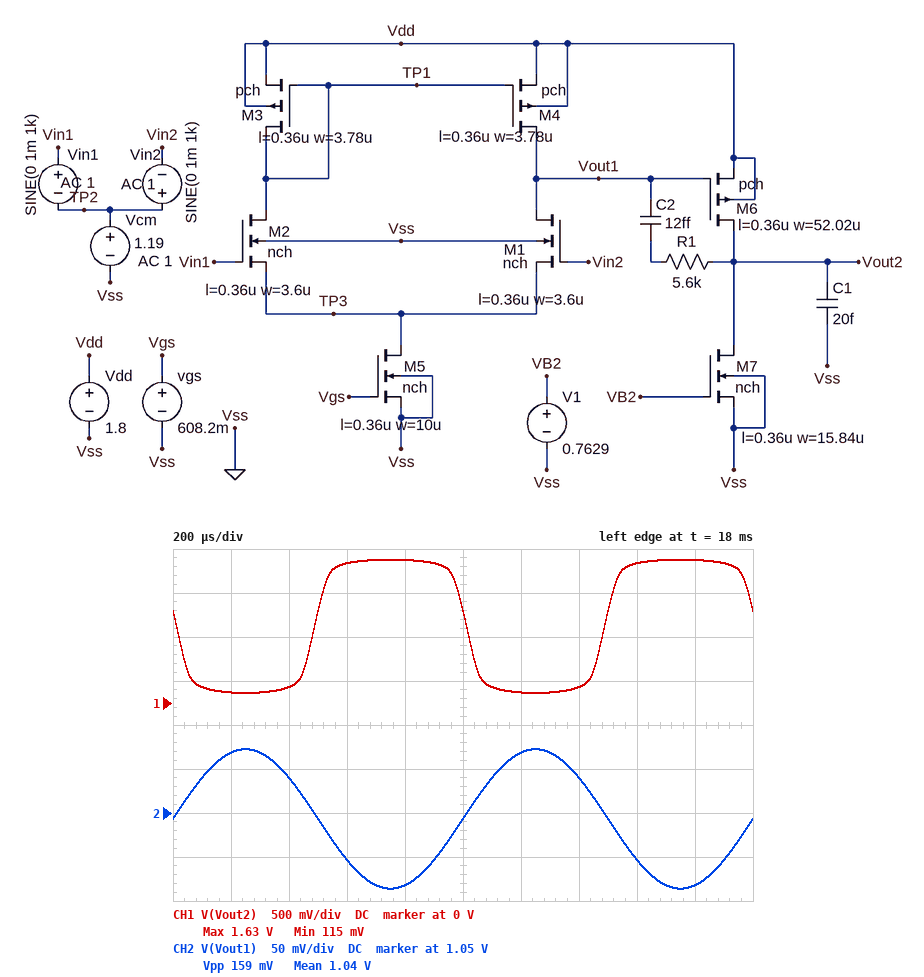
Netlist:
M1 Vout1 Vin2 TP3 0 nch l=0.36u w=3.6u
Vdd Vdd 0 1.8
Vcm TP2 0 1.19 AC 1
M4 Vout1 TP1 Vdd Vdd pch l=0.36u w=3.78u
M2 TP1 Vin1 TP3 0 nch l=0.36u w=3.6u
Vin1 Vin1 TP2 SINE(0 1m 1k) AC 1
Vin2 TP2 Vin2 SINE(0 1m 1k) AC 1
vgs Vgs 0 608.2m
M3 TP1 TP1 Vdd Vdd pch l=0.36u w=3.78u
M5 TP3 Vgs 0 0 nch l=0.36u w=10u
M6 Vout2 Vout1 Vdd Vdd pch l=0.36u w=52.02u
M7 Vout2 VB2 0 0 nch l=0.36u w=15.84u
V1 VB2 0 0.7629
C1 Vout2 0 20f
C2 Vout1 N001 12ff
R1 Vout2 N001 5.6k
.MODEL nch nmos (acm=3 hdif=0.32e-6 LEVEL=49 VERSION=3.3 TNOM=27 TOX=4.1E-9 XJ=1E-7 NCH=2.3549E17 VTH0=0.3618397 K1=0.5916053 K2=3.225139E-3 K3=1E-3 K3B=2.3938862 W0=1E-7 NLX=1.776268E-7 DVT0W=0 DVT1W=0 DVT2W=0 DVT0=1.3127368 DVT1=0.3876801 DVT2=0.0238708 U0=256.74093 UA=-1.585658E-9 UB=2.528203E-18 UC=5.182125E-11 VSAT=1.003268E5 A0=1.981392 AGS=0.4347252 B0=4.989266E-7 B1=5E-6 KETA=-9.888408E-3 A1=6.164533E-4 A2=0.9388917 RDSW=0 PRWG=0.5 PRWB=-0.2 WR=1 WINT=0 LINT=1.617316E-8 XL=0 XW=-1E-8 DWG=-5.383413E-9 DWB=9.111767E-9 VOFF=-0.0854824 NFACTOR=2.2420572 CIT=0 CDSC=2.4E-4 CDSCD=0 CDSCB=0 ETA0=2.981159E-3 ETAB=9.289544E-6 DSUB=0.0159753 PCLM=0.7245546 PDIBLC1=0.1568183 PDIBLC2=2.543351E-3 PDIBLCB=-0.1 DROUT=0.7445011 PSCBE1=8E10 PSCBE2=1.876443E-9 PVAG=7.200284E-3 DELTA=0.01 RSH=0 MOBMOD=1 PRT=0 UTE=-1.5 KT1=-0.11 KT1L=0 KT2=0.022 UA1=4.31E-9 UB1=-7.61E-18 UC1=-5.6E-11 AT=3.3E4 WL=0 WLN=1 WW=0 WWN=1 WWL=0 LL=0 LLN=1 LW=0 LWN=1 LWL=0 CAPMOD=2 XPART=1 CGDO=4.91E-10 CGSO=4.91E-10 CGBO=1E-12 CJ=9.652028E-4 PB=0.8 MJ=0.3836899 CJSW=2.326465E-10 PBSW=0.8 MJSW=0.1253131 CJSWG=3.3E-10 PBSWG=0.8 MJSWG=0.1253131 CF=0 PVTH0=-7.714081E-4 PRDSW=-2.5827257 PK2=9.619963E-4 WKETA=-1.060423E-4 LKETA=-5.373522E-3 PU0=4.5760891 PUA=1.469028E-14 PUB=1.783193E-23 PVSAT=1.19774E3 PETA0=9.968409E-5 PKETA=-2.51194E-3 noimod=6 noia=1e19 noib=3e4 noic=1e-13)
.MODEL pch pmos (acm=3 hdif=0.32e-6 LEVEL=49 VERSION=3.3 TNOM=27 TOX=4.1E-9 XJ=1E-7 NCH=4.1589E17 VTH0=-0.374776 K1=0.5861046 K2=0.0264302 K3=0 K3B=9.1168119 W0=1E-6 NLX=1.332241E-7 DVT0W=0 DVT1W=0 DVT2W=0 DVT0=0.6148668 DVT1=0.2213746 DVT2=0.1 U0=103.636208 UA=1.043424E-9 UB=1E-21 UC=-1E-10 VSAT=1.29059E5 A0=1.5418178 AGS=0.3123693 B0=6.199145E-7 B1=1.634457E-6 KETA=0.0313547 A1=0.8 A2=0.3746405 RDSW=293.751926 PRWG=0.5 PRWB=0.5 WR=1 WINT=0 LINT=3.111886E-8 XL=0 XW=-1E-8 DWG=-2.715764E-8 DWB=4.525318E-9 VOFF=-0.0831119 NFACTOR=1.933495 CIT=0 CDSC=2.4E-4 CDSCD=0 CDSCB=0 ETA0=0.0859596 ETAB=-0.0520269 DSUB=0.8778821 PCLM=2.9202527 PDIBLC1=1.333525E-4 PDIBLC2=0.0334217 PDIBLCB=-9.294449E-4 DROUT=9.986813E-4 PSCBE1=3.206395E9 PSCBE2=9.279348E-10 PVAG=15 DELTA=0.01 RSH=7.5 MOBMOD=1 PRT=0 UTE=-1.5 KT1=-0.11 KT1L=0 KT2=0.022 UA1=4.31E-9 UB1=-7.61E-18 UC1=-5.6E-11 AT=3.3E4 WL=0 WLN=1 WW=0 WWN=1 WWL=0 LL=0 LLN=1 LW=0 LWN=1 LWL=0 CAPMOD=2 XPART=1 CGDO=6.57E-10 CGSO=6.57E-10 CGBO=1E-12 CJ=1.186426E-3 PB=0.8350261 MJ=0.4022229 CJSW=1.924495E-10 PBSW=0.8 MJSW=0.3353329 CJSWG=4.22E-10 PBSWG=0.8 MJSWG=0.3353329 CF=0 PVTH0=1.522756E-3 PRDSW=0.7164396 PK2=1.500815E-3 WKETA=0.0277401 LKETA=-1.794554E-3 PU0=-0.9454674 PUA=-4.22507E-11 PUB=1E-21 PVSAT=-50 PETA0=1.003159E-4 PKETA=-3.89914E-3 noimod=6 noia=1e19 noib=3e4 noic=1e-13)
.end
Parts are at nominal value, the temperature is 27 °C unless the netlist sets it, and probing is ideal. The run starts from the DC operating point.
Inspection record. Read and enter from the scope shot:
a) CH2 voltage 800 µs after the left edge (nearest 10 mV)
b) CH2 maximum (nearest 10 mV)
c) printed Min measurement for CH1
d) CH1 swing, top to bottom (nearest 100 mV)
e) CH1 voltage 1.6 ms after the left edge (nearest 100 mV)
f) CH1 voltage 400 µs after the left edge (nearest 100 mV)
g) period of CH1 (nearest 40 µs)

970 mV
1.12 V
115 mV
1.5 V
1.6 V
200 mV
1.00 ms
